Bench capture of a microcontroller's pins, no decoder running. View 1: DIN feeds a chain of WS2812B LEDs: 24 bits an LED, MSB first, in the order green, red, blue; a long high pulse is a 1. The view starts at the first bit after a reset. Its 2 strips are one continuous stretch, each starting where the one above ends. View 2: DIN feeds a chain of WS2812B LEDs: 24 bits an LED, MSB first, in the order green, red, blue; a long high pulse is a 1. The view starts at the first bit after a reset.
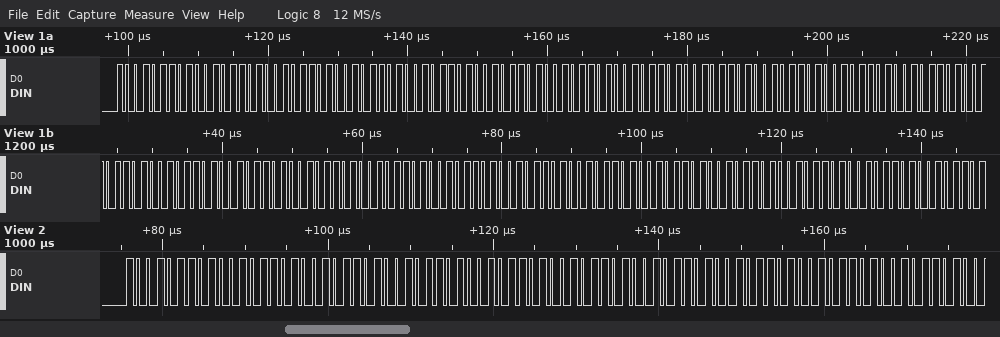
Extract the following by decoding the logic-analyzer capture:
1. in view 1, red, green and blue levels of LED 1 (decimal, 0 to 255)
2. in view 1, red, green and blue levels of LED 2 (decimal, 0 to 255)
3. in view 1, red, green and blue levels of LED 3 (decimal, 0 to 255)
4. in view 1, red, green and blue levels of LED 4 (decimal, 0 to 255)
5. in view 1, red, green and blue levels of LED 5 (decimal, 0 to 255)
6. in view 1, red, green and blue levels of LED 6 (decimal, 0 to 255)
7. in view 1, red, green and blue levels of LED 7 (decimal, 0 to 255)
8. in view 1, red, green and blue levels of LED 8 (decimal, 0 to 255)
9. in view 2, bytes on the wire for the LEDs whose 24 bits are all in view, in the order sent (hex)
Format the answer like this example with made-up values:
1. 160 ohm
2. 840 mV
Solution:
1. 150, 150, 150
2. 150, 150, 150
3. 150, 150, 150
4. 150, 150, 150
5. 150, 150, 150
6. 150, 150, 150
7. 150, 150, 150
8. 150, 150, 150
9. 96 96 96 96 96 96 96 96 96
